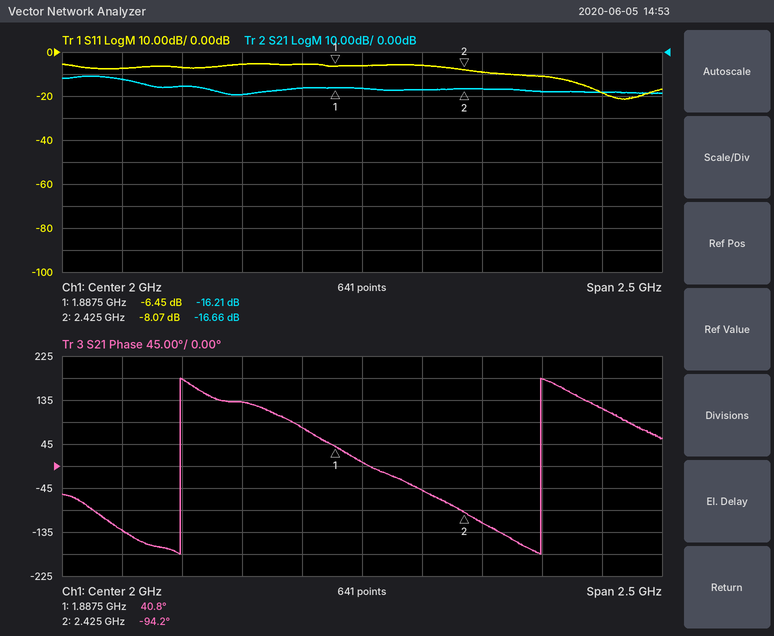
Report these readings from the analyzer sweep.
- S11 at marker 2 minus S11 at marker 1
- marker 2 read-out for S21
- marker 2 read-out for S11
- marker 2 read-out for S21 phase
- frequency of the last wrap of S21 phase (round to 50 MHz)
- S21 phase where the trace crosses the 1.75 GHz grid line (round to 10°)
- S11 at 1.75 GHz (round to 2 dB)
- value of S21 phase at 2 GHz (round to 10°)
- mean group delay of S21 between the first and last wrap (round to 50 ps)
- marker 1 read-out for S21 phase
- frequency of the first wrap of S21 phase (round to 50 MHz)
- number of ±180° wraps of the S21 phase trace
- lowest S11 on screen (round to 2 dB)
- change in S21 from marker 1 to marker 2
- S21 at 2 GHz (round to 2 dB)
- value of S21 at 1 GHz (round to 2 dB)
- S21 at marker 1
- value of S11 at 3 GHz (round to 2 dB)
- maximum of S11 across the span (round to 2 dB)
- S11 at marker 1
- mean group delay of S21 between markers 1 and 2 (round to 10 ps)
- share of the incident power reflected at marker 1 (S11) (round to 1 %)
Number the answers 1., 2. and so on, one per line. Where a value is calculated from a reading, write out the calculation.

1. -8.07 − (-6.45) = -1.62 dB
2. -16.66 dB
3. -8.07 dB
4. -94.2°
5. 2.75 GHz
6. 80°
7. -6 dB
8. 10°
9. 1 cycle / (2.75 GHz − 1.25 GHz) ≈ 667 ps, so 650 ps to the nearest 50 ps
10. 40.8°
11. 1.25 GHz
12. 2
13. -22 dB
14. -16.66 − (-16.21) = -0.45 dB
15. -16 dB
16. -12 dB
17. -16.21 dB
18. -18 dB
19. -6 dB
20. -6.45 dB
21. −(-94.2° − (40.8°))/(360° × 537.5 MHz) ≈ 698 ps, so 700 ps to the nearest 10 ps
22. 10^(-6.45/10) ≈ 23 %
